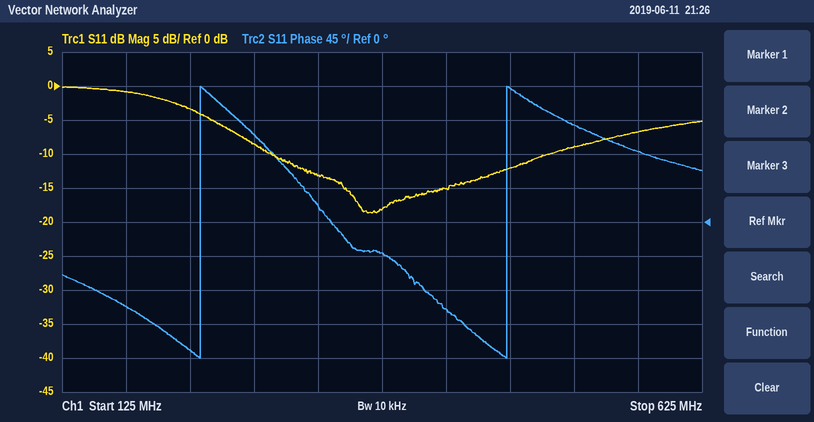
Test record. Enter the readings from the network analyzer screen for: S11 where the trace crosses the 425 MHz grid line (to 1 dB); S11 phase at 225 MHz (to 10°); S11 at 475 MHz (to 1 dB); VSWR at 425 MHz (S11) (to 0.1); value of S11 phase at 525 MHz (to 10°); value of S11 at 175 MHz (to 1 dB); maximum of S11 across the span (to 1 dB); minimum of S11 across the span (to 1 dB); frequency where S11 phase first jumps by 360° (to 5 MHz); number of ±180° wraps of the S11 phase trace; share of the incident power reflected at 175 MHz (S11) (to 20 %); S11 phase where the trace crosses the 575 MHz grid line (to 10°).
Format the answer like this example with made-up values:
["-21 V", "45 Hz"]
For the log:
["-15 dB", "-170°", "-12 dB", "1.4", "130°", "-1 dB", "0 dB", "-19 dB", "235 MHz", "2", "80 %", "90°"]
